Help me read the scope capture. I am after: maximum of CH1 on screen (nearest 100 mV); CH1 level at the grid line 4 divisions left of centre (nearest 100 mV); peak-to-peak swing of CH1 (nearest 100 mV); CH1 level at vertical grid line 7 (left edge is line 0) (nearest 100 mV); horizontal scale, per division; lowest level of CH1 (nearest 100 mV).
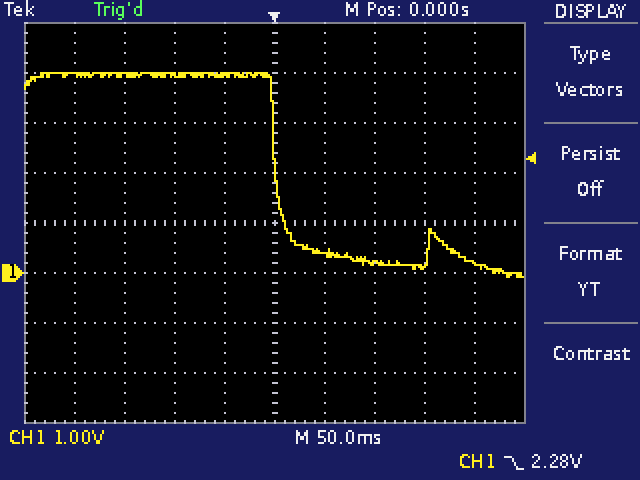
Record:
4.0 V
4.0 V
4.1 V
200 mV
50 ms
-100 mV
